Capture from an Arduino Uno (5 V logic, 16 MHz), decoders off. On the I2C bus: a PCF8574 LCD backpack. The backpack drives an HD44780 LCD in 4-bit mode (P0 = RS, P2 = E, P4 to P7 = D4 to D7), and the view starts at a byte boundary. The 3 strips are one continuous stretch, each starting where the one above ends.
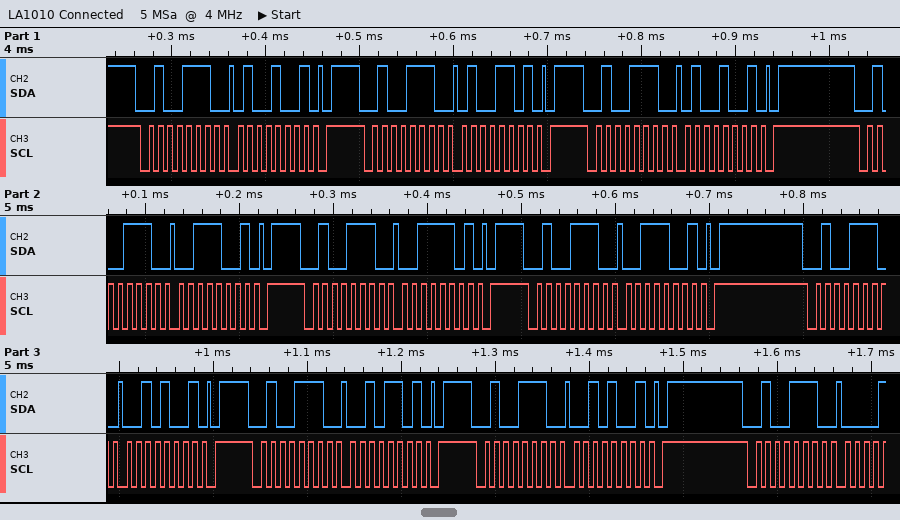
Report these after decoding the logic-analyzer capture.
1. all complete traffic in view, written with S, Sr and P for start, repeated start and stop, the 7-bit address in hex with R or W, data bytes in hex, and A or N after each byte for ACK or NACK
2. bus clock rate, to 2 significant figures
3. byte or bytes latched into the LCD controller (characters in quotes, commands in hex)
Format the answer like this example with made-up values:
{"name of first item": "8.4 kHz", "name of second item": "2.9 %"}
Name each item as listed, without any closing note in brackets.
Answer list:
{"all complete traffic in view, written with S, Sr and P for start, repeated start and stop, the 7-bit address in hex with R or W, data bytes in hex, and A or N after each byte for ACK or NACK": "S 27W A 49 A P S 27W A 4D A P S 27W A 49 A P S 27W A 39 A P S 27W A 3D A P S 27W A 39 A P S 27W A 29 A P S 27W A 2D A P S 27W A 29 A P S 27W A", "bus clock rate, to 2 significant figures": "100 kHz", "byte or bytes latched into the LCD controller": "'C'"}
